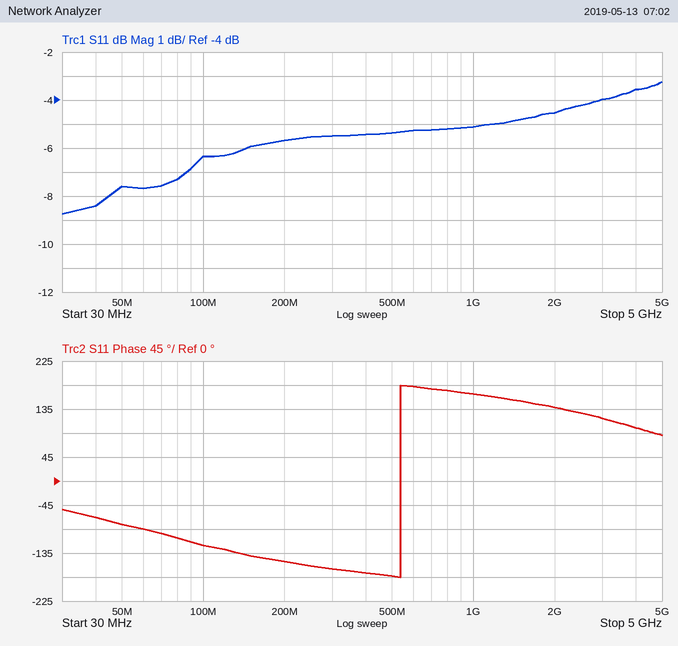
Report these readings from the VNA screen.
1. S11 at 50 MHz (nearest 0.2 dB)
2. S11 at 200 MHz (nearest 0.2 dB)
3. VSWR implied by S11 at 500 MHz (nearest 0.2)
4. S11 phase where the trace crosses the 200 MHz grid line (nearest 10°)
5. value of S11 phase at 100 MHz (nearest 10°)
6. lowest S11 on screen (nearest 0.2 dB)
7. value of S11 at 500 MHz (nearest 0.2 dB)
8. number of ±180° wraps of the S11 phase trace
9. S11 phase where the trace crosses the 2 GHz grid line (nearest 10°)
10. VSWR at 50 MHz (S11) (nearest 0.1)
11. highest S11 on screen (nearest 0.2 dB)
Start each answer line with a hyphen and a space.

- -7.6 dB
- -5.6 dB
- 3.4
- -150°
- -120°
- -8.8 dB
- -5.4 dB
- 1
- 140°
- 2.4
- -3.2 dB
